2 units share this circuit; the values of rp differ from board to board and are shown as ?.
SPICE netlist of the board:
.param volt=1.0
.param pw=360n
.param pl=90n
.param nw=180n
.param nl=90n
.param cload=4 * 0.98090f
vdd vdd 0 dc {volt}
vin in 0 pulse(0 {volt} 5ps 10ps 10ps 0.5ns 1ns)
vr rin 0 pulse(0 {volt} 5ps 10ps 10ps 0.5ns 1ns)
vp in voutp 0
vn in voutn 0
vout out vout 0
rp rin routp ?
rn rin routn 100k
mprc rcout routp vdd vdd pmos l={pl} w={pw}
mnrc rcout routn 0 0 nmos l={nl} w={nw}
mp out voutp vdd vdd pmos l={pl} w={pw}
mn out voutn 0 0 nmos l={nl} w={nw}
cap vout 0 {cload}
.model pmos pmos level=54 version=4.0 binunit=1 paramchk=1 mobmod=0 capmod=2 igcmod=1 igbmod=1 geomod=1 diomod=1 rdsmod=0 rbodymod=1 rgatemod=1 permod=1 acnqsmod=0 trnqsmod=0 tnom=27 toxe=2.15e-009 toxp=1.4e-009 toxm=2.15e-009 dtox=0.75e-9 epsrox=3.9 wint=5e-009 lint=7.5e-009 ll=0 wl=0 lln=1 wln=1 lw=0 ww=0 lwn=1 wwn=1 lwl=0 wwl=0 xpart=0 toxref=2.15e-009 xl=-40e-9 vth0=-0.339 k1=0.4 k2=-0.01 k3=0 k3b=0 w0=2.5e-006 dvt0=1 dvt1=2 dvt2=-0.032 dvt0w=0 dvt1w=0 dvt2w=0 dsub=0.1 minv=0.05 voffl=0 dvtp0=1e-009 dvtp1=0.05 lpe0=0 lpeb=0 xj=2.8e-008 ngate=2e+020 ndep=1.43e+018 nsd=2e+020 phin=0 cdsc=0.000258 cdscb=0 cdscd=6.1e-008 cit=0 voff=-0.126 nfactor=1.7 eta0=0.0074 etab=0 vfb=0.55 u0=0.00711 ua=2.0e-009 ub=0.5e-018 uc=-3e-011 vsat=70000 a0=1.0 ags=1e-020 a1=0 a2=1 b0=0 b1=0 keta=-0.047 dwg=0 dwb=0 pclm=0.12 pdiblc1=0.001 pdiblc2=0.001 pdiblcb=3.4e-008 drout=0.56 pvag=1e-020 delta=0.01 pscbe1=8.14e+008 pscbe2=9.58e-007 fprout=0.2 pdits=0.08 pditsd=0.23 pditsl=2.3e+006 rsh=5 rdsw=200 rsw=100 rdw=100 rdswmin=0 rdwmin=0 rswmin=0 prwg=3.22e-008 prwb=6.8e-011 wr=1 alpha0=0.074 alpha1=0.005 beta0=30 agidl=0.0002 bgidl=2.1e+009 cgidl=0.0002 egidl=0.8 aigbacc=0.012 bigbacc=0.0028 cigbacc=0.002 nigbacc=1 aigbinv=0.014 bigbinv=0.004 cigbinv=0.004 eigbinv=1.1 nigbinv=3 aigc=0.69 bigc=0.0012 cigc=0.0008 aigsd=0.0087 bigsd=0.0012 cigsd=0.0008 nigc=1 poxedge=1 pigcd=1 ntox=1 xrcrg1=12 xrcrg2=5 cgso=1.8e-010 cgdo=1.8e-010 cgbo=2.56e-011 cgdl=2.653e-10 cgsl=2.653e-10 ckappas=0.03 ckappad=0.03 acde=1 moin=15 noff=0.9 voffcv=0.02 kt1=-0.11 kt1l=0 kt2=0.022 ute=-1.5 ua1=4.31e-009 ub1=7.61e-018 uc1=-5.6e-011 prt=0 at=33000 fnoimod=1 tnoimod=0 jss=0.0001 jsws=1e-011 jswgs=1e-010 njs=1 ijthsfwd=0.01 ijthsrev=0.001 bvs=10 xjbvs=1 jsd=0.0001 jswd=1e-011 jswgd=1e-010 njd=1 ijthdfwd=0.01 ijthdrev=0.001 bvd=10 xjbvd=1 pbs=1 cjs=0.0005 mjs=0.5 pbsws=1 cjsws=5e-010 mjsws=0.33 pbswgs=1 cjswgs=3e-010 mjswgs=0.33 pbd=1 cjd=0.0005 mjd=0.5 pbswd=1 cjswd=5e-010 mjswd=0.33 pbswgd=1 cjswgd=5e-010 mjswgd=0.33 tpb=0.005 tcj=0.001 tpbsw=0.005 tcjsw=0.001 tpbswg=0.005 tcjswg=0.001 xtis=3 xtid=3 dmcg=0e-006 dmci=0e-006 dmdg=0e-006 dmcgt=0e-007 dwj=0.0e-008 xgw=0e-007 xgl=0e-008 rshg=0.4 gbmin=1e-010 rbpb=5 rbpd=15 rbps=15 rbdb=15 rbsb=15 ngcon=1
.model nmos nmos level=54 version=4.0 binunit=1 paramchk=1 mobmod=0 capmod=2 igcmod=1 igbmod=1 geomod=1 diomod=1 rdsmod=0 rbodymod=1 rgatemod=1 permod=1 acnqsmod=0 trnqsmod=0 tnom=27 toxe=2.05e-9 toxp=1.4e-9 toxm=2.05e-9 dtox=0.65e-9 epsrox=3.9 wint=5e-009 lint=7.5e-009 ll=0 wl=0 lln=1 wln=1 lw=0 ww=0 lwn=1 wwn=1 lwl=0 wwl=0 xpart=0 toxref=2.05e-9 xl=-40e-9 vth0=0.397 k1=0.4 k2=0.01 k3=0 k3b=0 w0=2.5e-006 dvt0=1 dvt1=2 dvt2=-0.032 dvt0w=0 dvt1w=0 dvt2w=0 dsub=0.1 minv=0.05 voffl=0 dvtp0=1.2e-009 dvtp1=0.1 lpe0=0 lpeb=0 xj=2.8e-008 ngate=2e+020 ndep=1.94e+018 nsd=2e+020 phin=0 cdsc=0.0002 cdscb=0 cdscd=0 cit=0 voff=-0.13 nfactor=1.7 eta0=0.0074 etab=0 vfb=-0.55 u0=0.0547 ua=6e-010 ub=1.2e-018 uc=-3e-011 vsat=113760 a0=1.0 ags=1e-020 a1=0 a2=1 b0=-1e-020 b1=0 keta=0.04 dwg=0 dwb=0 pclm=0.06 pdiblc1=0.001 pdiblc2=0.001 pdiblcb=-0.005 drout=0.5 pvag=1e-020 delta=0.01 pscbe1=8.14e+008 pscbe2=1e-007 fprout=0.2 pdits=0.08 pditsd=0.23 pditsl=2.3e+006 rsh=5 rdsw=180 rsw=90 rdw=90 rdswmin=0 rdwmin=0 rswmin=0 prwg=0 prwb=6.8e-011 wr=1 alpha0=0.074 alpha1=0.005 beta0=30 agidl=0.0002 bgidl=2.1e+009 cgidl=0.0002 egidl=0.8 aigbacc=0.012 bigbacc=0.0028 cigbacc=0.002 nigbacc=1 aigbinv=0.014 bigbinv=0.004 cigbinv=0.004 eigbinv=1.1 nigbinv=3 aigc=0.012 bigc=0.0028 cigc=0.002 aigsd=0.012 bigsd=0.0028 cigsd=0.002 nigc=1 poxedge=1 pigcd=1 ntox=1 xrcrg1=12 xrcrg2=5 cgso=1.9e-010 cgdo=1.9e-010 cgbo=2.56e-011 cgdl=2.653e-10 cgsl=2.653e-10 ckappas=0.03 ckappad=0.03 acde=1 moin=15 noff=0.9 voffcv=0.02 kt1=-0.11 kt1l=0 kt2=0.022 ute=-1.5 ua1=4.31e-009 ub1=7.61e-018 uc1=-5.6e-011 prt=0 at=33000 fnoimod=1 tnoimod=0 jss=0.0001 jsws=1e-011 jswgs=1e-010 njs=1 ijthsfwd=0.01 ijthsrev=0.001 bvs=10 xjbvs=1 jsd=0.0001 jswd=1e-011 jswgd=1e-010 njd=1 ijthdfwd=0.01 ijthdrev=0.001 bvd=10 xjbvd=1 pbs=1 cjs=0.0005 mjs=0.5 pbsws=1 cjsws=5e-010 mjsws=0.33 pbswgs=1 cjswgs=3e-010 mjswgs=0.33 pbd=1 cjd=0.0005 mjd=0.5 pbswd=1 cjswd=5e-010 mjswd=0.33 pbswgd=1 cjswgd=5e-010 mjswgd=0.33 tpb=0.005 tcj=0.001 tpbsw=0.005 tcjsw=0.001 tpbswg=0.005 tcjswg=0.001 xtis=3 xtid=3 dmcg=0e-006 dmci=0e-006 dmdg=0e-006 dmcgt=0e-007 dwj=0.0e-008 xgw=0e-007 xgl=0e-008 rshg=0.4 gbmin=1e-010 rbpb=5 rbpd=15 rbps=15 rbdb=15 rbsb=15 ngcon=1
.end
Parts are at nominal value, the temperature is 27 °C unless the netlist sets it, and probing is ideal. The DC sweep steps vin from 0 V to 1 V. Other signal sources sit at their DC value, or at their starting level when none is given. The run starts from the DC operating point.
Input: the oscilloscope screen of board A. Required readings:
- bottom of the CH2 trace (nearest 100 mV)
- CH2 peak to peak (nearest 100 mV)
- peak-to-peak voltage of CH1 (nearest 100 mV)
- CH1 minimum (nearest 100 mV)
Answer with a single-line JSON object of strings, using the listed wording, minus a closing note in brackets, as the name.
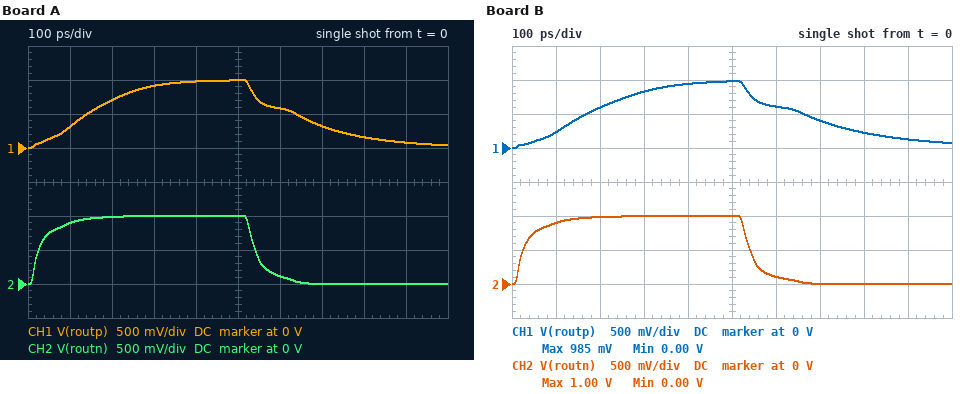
{"bottom of the CH2 trace": "0 V", "CH2 peak to peak": "1.0 V", "peak-to-peak voltage of CH1": "1.0 V", "CH1 minimum": "0 V"}
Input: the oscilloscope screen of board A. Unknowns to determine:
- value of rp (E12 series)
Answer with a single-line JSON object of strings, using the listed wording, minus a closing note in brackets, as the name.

{"value of rp": "220 kΩ"}
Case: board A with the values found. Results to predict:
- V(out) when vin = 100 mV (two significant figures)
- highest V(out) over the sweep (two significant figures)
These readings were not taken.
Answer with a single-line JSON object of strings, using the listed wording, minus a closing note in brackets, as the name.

{"V(out) when vin = 100 mV": "1.0 V", "highest V(out) over the sweep": "1.0 V"}
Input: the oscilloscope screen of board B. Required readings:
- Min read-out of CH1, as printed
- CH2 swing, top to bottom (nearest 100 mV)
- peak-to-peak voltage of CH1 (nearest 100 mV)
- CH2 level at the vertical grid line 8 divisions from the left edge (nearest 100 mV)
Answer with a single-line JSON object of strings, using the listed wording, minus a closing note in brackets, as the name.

{"Min read-out of CH1, as printed": "0.00 V", "CH2 swing, top to bottom": "1.0 V", "peak-to-peak voltage of CH1": "1.0 V", "CH2 level at the vertical grid line 8 divisions from the left edge": "0 V"}
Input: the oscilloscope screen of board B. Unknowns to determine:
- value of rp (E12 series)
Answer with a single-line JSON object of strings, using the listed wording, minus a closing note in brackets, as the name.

{"value of rp": "270 kΩ"}
